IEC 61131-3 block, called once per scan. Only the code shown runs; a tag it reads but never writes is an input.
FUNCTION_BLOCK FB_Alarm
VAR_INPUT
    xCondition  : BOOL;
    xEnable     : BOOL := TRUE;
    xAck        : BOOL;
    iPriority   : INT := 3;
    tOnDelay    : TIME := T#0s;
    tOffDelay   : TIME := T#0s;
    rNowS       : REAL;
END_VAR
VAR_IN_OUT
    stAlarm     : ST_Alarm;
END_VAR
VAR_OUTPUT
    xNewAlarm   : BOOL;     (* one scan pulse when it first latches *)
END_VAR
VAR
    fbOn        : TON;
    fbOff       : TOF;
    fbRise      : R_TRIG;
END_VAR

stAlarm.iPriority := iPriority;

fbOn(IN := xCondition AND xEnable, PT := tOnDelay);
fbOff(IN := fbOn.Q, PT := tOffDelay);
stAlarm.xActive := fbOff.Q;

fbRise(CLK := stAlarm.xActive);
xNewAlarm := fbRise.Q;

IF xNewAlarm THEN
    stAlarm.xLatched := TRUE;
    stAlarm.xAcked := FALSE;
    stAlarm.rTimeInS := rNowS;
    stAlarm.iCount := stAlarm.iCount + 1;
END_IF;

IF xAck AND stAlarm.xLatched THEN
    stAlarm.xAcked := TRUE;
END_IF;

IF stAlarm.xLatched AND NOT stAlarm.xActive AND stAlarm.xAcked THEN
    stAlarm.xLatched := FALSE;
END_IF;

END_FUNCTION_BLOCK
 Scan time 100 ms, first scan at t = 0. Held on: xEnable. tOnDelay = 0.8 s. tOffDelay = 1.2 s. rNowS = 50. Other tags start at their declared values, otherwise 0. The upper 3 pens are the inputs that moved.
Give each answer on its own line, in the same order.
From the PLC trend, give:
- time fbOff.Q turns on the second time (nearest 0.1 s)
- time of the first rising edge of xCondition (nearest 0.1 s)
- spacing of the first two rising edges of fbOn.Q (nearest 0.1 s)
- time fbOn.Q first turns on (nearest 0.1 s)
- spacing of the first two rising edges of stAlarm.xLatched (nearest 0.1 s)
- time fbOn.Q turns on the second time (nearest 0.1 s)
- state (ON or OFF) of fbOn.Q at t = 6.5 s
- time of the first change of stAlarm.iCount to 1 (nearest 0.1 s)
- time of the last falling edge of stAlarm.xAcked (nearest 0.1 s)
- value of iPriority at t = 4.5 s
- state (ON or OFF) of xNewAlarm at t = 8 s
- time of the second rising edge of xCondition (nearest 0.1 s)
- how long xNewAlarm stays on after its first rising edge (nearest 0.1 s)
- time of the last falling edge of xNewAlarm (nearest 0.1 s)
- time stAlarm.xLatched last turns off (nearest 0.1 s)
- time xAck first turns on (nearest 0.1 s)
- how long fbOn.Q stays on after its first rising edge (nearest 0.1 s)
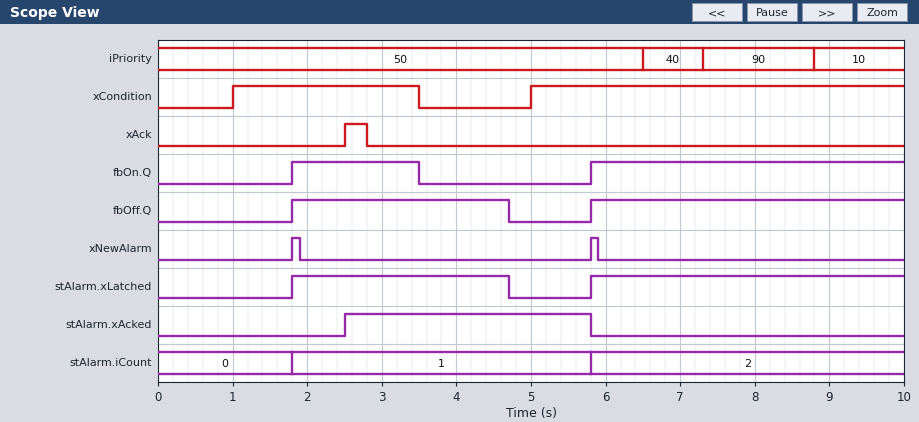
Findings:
5.8 s
1.0 s
4.0 s
1.8 s
4.0 s
5.8 s
ON
1.8 s
5.8 s
50
OFF
5.0 s
0.1 s
5.9 s
4.7 s
2.5 s
1.7 s
